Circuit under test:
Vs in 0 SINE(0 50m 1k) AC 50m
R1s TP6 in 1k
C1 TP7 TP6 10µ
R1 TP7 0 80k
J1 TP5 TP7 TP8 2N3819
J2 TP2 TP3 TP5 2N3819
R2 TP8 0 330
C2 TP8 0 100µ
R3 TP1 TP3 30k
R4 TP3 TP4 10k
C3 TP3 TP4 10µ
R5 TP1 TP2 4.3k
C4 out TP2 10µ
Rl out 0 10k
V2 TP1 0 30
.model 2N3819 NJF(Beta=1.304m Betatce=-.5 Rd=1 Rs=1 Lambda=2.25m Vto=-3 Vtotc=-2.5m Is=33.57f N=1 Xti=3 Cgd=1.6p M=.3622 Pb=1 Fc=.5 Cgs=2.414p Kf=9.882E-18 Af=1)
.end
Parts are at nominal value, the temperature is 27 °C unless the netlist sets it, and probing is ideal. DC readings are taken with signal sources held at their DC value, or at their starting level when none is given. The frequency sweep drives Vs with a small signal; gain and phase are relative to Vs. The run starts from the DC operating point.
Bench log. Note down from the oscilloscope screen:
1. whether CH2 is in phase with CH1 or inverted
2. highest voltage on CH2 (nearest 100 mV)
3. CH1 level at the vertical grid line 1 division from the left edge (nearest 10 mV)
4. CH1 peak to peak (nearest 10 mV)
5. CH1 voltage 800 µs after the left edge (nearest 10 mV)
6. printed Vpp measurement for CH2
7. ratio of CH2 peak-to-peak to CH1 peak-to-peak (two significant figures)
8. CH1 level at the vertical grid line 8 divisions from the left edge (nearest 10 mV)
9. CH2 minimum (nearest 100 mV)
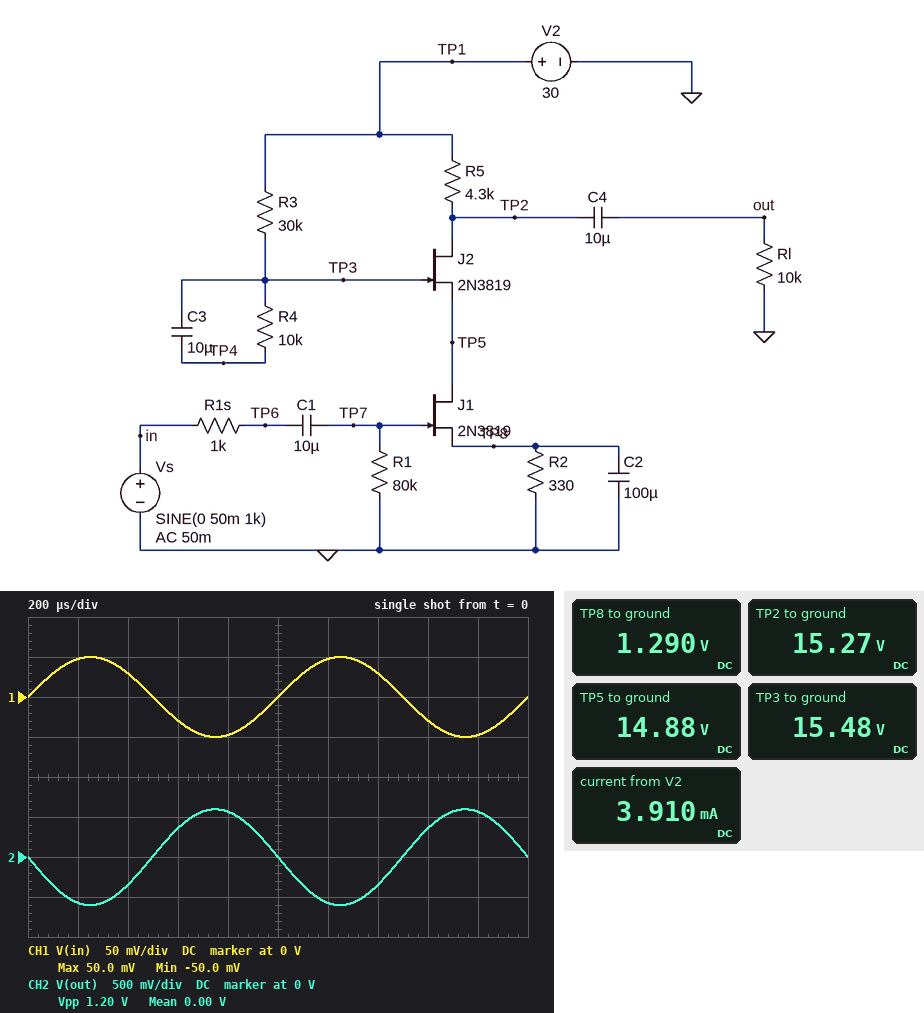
inverted
600 mV
50 mV
100 mV
-50 mV
1.20 V
12
-30 mV
-600 mV
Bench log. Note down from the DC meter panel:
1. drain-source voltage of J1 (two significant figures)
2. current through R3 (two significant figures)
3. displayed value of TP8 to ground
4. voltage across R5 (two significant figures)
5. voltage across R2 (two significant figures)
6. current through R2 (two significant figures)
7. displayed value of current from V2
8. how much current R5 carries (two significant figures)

14 V
480 µA
1.290 V
15 V
1.3 V
3.9 mA
3.910 mA
3.4 mA
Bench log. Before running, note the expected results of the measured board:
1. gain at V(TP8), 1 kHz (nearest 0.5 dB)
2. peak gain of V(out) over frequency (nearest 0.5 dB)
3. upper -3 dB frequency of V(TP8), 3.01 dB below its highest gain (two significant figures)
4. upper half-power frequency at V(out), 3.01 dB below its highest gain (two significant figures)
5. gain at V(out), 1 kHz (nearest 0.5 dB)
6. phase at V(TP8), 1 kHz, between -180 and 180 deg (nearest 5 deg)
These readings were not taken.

-43.0 dB
21.5 dB
12 Hz
20 MHz
21.5 dB
-90 deg
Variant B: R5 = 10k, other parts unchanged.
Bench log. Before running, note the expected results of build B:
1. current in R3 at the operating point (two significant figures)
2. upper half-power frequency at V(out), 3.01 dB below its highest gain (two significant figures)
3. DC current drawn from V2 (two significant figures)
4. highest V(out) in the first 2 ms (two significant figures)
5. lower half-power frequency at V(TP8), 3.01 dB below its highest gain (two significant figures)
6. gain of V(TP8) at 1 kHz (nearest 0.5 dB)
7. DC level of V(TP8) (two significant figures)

900 µA
40 MHz
3.6 mA
82 mV
370 mHz
-65.5 dB
1.2 V
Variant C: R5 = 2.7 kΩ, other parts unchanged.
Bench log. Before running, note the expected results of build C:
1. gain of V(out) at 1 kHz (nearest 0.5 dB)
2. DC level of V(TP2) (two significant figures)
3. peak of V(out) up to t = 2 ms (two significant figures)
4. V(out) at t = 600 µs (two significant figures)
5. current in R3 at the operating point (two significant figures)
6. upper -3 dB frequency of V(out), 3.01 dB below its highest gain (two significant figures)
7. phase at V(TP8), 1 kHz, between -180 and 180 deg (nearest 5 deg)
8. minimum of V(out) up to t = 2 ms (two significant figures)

19.0 dB
20 V
440 mV
260 mV
320 µA
28 MHz
-90 deg
-440 mV
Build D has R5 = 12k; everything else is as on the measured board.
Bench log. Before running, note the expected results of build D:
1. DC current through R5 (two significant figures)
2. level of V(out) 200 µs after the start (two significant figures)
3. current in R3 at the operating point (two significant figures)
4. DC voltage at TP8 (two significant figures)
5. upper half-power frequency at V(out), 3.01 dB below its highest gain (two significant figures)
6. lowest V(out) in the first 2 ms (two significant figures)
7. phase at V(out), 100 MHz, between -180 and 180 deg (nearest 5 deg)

2.3 mA
-30 mV
920 µA
1.1 V
48 MHz
-31 mV
95 deg
